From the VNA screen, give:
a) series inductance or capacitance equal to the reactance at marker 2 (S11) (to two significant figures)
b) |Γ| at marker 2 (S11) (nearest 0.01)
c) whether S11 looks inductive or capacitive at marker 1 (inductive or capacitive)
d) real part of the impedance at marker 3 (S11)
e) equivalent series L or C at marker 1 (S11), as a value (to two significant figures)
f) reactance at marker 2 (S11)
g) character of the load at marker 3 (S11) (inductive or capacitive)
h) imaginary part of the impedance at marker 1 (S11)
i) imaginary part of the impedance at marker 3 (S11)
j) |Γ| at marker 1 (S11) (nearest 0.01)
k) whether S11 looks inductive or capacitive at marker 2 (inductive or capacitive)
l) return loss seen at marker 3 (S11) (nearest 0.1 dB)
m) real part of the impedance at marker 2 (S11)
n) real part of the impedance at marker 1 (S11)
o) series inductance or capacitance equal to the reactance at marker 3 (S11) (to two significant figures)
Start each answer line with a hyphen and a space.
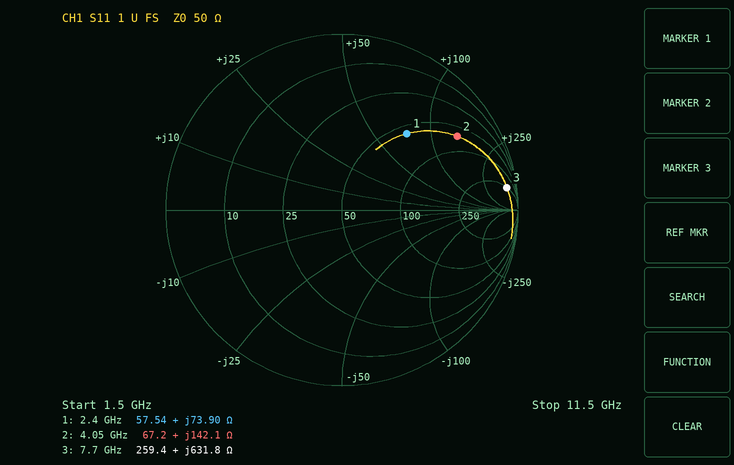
- 5.6 nH
- 0.78
- inductive
- 259.4 Ω
- 4.9 nH
- +142.1 Ω
- inductive
- +73.90 Ω
- +631.8 Ω
- 0.57
- inductive
- 0.5 dB
- 67.2 Ω
- 57.54 Ω
- 13 nH
